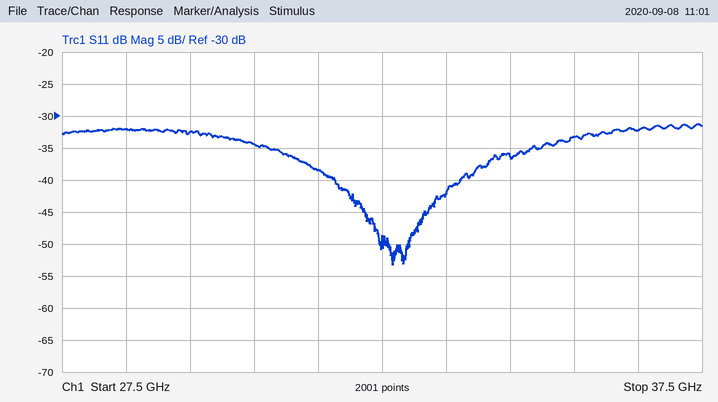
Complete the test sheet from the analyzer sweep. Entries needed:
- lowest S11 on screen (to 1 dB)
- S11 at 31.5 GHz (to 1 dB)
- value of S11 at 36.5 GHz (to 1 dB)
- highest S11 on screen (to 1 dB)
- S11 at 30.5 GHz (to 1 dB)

-53 dB
-38 dB
-32 dB
-31 dB
-34 dB
